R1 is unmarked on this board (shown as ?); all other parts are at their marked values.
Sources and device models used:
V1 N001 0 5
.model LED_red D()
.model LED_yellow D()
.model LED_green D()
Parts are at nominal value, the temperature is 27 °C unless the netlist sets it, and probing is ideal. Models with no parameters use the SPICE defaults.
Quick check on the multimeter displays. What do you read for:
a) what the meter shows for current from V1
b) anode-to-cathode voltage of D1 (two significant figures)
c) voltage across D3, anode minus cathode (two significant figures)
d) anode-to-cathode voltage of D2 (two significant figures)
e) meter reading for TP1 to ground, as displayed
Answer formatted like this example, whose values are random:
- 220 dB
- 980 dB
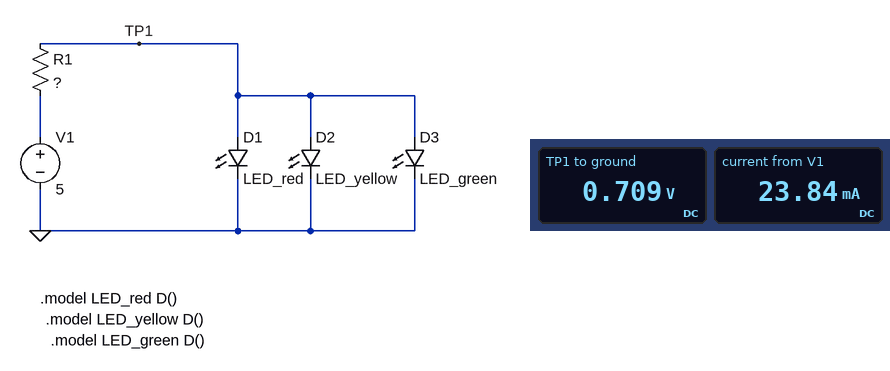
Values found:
- 23.84 mA
- 710 mV
- 710 mV
- 710 mV
- 0.709 V
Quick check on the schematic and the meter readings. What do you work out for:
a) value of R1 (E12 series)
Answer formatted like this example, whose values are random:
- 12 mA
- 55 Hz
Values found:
- 180 Ω
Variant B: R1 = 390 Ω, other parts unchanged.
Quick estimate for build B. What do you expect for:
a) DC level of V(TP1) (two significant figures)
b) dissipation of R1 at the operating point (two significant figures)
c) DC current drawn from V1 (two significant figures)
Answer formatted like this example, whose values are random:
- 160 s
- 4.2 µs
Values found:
- 690 mV
- 48 mW
- 11 mA
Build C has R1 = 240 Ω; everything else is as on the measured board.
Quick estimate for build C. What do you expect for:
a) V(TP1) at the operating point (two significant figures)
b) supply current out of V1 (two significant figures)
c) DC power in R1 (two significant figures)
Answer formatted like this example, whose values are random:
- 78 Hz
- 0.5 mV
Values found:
- 700 mV
- 18 mA
- 77 mW
